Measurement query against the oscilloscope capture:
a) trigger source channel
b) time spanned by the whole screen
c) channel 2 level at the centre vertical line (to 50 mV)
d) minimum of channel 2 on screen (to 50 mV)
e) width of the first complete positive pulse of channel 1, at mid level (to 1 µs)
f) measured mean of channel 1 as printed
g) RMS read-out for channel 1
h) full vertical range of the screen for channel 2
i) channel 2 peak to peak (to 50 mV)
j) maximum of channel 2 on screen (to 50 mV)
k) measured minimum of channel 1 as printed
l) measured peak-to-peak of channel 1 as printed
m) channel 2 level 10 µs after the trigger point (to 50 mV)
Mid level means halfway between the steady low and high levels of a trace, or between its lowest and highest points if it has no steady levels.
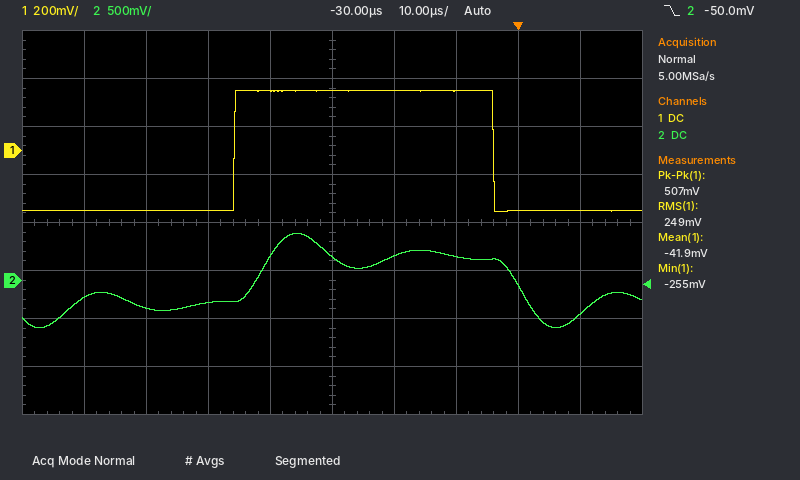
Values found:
channel 2
100 µs
250 mV
-500 mV
42 µs
-41.9 mV
249 mV
4 V
1.00 V
500 mV
-255 mV
507 mV
-350 mV
